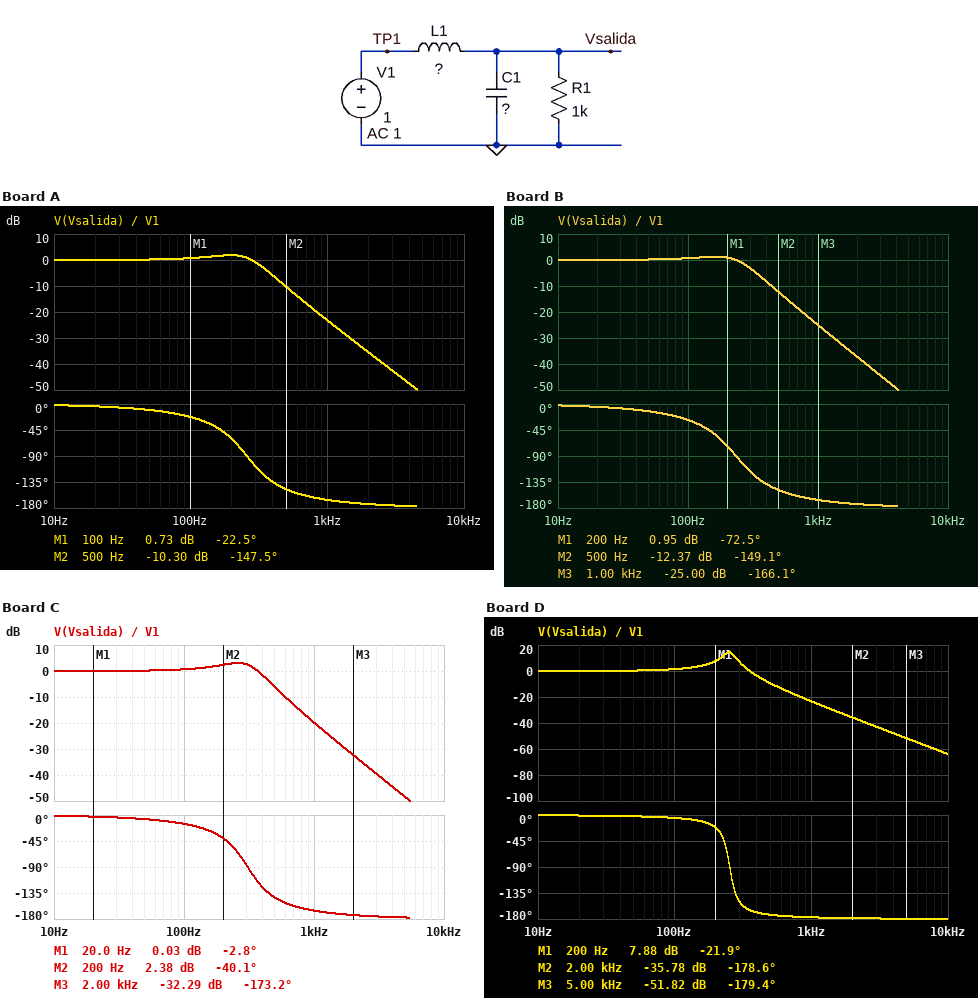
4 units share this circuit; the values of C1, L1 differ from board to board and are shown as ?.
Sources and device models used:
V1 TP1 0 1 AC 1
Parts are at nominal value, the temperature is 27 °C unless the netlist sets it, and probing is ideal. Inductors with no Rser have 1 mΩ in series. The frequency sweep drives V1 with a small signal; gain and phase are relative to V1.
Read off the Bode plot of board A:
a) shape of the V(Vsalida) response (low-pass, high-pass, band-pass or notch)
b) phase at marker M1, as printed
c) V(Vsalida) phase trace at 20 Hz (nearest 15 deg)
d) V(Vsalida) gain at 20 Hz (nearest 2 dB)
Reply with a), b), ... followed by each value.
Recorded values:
a) low-pass
b) -22.5 deg
c) 0 deg
d) 0 dB
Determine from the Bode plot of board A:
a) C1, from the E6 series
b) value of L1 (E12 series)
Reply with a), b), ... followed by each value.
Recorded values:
a) 680 nF
b) 560 mH
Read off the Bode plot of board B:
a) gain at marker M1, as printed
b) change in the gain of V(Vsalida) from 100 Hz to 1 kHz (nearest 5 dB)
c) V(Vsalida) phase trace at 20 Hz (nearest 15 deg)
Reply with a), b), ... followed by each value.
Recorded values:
a) 0.95 dB
b) -25 dB
c) 0 deg
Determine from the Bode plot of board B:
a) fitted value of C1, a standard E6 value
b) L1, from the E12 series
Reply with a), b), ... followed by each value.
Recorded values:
a) 680 nF
b) 680 mH
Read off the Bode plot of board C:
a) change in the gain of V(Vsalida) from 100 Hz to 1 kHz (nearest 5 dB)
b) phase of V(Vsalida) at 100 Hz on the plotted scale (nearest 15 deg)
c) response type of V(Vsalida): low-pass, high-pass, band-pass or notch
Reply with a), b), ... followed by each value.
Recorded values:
a) -20 dB
b) -15 deg
c) low-pass
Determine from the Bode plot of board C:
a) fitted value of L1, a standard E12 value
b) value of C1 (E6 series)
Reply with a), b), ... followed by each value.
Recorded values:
a) 390 mH
b) 680 nF
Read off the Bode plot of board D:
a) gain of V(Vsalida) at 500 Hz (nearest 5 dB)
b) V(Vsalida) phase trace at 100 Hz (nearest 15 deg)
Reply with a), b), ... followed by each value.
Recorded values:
a) -10 dB
b) 0 deg
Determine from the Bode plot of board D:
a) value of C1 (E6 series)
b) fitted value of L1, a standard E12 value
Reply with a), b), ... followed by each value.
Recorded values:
a) 3.3 µF
b) 120 mH
